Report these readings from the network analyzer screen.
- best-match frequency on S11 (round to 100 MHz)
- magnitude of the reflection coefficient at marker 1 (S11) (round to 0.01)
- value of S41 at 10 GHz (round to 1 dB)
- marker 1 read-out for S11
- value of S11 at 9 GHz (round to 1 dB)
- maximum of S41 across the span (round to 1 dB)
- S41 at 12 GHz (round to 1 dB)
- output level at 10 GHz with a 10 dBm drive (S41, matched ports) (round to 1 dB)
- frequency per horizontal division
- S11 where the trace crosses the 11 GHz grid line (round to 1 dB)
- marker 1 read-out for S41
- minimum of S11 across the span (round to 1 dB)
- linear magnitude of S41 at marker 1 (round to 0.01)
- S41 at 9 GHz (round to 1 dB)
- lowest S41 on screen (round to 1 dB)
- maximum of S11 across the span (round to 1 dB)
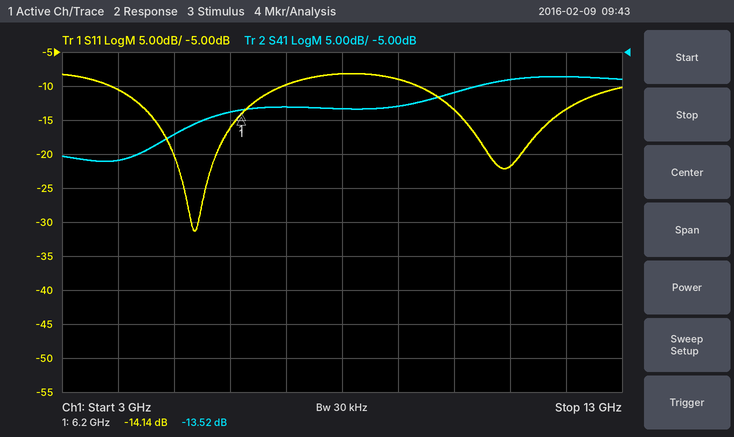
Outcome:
5.4 GHz
0.20
-11 dB
-14.14 dB
-9 dB
-9 dB
-9 dB
-1 dBm
1 GHz
-22 dB
-13.52 dB
-31 dB
0.21
-13 dB
-21 dB
-8 dB
